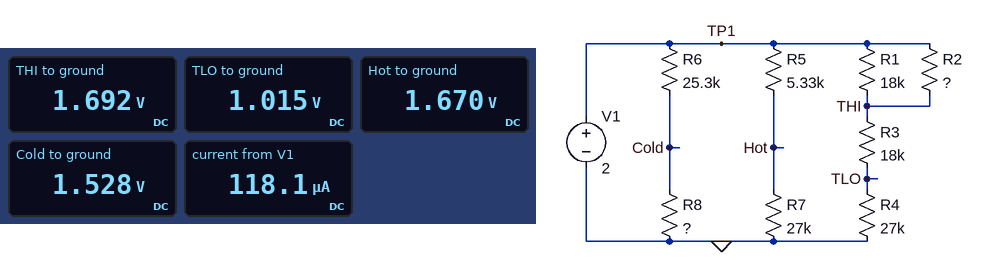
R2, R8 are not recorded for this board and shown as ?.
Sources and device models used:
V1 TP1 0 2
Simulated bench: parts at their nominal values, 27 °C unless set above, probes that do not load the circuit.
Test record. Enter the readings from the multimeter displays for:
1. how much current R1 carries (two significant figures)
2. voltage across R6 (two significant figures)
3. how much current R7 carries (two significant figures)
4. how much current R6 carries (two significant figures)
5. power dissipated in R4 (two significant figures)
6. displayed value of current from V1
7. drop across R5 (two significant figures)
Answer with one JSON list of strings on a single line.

["17 µA", "470 mV", "62 µA", "19 µA", "38 µW", "118.1 µA", "330 mV"]
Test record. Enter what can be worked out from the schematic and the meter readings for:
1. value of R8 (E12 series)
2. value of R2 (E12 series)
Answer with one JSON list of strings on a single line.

["82 kΩ", "15 kΩ"]
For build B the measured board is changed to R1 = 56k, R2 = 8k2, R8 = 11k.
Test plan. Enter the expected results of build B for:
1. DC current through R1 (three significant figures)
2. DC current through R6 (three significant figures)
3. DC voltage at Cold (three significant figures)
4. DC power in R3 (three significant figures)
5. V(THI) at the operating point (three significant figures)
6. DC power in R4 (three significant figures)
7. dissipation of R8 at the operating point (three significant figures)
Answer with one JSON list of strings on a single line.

["4.90 µA", "55.1 µA", "606 mV", "26.5 µW", "1.73 V", "39.7 µW", "33.4 µW"]
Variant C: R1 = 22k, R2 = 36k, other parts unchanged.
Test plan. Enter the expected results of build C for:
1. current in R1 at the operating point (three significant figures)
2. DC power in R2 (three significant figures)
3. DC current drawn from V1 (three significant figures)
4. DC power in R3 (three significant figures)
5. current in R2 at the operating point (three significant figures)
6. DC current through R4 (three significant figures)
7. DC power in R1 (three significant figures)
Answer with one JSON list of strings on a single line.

["21.2 µA", "6.02 µW", "115 µA", "20.9 µW", "12.9 µA", "34.1 µA", "9.85 µW"]
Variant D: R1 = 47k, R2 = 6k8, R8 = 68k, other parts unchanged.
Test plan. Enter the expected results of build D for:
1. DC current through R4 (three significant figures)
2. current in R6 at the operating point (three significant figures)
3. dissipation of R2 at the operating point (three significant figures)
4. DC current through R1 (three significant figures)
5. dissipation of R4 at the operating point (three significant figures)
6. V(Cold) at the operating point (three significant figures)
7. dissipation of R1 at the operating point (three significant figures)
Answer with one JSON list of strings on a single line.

["39.3 µA", "21.4 µA", "8.00 µW", "4.96 µA", "41.6 µW", "1.46 V", "1.16 µW"]
